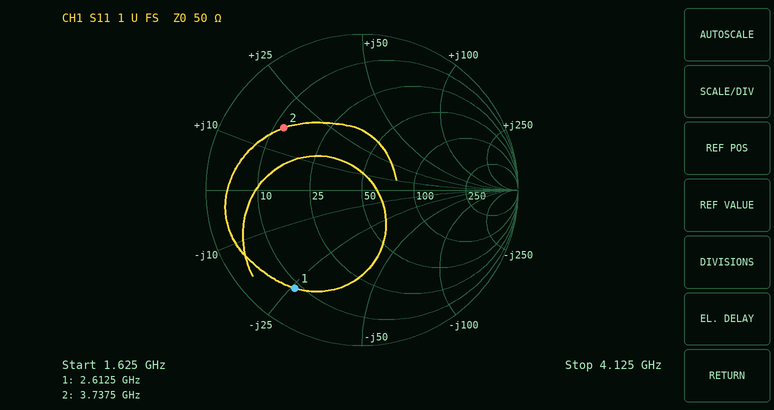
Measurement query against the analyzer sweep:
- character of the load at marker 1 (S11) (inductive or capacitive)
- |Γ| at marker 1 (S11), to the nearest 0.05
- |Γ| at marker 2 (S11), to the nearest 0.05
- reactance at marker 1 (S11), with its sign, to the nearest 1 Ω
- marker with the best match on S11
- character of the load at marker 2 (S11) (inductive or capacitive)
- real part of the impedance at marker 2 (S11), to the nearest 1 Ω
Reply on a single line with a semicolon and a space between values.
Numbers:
capacitive; 0.75; 0.65; -26 Ω; marker 2; inductive; 12 Ω
